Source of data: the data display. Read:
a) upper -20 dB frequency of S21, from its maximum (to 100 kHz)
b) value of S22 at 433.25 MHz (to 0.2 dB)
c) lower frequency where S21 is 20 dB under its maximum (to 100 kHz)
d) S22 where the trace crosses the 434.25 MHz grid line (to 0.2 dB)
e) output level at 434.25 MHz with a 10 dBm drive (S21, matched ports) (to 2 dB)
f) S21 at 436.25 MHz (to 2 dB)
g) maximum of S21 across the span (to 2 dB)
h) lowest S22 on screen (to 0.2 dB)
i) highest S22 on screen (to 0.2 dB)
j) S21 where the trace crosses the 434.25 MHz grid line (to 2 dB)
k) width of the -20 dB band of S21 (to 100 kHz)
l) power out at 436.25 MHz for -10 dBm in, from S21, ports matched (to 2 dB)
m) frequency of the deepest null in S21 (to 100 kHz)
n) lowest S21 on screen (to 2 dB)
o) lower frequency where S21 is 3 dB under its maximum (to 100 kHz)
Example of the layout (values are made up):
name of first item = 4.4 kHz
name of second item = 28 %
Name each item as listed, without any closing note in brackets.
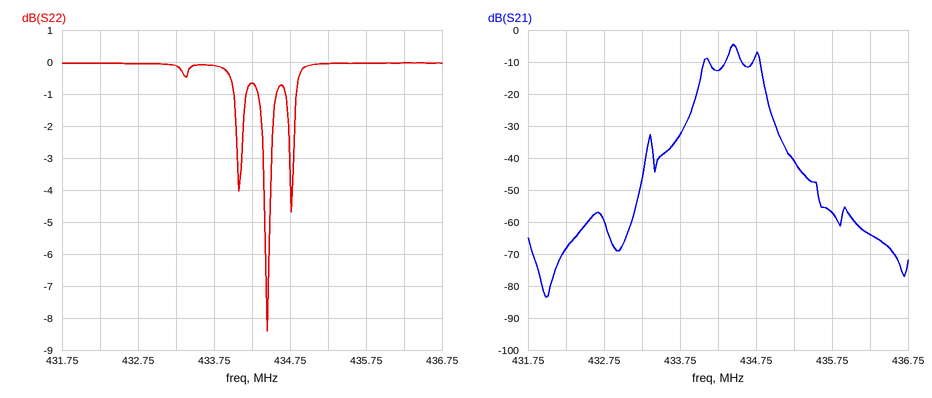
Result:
upper -20 dB frequency of S21, from its maximum = 434.9 MHz
value of S22 at 433.25 MHz = -0.2 dB
lower frequency where S21 is 20 dB under its maximum = 433.9 MHz
S22 where the trace crosses the 434.25 MHz grid line = -0.6 dB
output level at 434.25 MHz with a 10 dBm drive (S21, matched ports) = -2 dBm
S21 at 436.25 MHz = -64 dB
maximum of S21 across the span = -4 dB
lowest S22 on screen = -8.4 dB
highest S22 on screen = 0.0 dB
S21 where the trace crosses the 434.25 MHz grid line = -12 dB
width of the -20 dB band of S21 = 1.0 MHz
power out at 436.25 MHz for -10 dBm in, from S21, ports matched = -74 dBm
frequency of the deepest null in S21 = 432.0 MHz
lowest S21 on screen = -84 dB
lower frequency where S21 is 3 dB under its maximum = 434.4 MHz
